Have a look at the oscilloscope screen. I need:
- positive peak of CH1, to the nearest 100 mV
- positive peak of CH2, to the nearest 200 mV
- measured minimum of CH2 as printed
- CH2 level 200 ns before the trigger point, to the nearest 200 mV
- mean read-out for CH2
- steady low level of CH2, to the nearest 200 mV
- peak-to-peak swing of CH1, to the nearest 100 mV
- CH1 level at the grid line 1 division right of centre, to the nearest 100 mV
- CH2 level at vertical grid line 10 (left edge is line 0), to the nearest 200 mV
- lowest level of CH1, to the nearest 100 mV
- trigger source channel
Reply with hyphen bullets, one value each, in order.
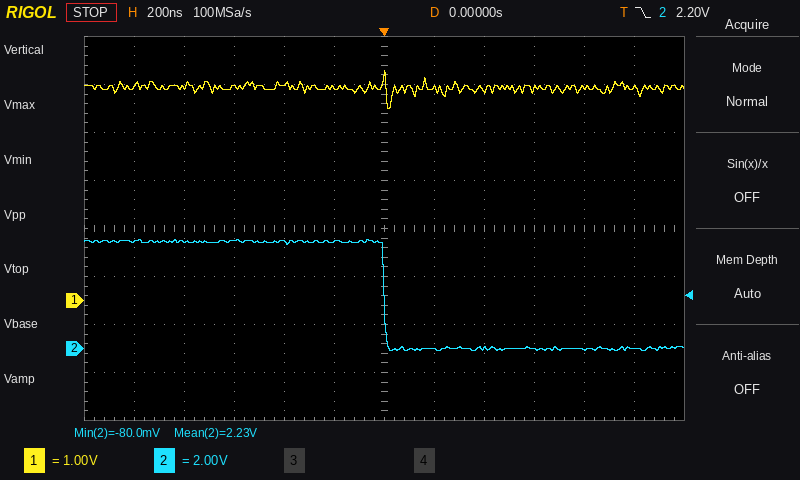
- 4.8 V
- 4.6 V
- -80.0 mV
- 4.4 V
- 2.23 V
- 0.0 V
- 800 mV
- 4.4 V
- 0.0 V
- 4.0 V
- CH2
